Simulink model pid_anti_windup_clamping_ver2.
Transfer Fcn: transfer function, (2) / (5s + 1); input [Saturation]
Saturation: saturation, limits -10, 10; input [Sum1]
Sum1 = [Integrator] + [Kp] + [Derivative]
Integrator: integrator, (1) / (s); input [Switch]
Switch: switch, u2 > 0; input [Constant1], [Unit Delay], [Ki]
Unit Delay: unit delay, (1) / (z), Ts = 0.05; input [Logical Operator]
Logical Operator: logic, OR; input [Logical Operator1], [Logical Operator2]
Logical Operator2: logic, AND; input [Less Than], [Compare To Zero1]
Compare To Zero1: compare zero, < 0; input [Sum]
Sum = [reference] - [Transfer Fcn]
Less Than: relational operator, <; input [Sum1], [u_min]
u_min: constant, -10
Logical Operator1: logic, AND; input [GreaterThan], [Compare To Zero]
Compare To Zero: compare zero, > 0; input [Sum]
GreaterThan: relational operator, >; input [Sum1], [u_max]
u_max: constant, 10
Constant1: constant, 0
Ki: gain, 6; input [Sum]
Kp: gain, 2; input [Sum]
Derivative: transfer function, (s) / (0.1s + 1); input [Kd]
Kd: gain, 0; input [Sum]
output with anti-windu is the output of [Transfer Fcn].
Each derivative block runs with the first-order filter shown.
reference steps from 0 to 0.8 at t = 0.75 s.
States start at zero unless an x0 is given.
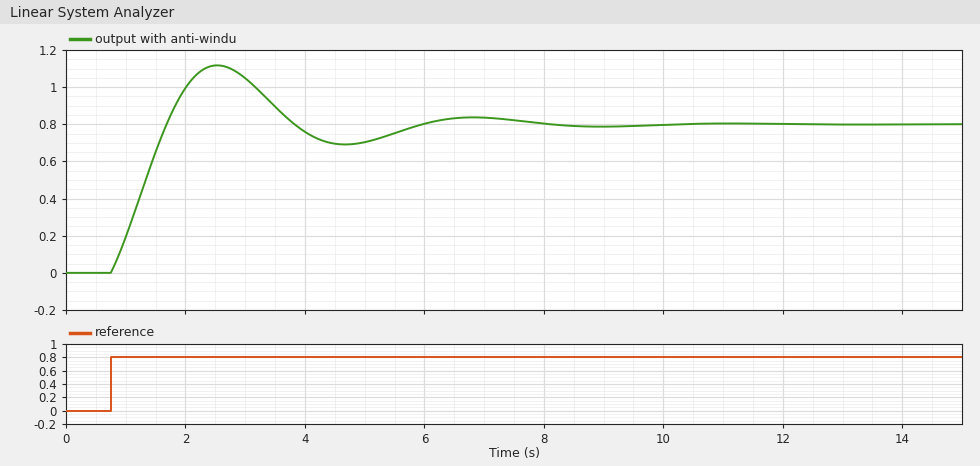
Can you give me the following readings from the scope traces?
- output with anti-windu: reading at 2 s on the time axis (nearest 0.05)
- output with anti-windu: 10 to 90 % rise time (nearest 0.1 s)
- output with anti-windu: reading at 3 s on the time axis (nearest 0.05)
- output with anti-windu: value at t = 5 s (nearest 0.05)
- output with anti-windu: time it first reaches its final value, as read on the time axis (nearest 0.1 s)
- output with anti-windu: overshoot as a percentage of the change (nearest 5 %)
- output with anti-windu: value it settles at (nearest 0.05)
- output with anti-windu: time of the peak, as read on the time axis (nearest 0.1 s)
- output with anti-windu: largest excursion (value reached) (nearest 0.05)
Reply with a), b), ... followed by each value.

a) 1.00
b) 0.7 s
c) 1.05
d) 0.70
e) 1.7 s
f) 40 %
g) 0.80
h) 2.5 s
i) 1.10
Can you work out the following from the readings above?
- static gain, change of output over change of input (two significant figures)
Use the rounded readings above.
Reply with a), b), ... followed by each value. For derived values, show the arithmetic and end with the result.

a) (0.8 - 0) / (0.8 - 0) = 1.0
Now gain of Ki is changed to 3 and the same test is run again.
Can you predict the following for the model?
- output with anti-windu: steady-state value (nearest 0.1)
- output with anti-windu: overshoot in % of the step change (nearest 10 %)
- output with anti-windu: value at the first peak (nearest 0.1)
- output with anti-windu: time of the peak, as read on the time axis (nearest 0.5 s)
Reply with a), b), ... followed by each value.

a) 0.8
b) 30 %
c) 1.0
d) 3.0 s
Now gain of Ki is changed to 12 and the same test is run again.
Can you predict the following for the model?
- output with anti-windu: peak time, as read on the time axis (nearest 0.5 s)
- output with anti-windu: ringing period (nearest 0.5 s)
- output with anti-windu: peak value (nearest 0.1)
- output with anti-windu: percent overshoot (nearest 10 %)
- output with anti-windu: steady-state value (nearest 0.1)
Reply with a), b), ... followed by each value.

a) 2.0 s
b) 3.0 s
c) 1.2
d) 50 %
e) 0.8
